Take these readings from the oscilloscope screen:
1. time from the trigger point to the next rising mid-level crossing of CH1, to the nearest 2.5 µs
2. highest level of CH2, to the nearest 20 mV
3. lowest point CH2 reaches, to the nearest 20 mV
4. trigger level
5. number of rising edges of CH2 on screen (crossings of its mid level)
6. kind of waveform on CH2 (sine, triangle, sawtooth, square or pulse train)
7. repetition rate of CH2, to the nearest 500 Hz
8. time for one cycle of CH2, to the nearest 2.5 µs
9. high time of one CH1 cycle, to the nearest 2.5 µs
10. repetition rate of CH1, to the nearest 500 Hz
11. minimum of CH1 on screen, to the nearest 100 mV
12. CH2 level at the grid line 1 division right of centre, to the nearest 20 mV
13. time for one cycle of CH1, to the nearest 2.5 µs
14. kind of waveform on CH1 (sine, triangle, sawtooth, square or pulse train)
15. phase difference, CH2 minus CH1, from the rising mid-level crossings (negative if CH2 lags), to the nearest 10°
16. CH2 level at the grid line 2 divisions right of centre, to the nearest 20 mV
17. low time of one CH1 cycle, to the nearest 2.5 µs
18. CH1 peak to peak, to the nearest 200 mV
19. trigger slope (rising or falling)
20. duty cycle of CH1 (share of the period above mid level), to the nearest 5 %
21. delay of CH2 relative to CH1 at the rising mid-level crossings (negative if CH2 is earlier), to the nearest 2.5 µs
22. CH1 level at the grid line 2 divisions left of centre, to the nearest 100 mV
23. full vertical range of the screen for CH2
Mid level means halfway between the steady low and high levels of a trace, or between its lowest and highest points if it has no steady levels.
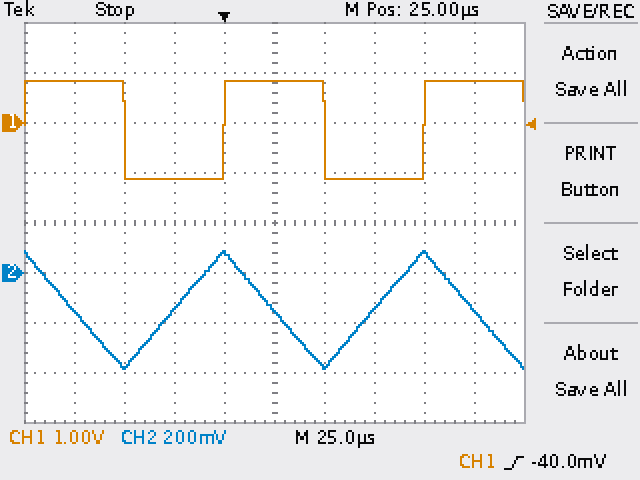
100.0 µs
80 mV
-380 mV
-40.0 mV
2
triangle
10.0 kHz
100.0 µs
50.0 µs
10.0 kHz
-1.1 V
-380 mV
100.0 µs
square
+90°
-140 mV
50.0 µs
2.0 V
rising
50 %
-25.0 µs
-1.1 V
1.6 V
